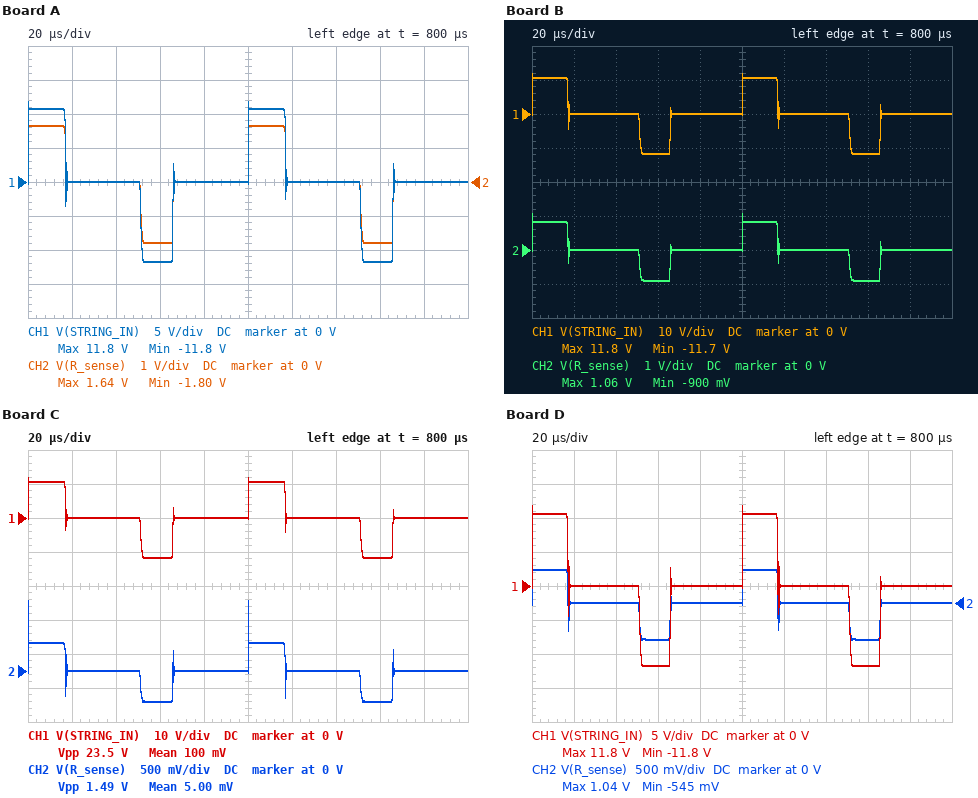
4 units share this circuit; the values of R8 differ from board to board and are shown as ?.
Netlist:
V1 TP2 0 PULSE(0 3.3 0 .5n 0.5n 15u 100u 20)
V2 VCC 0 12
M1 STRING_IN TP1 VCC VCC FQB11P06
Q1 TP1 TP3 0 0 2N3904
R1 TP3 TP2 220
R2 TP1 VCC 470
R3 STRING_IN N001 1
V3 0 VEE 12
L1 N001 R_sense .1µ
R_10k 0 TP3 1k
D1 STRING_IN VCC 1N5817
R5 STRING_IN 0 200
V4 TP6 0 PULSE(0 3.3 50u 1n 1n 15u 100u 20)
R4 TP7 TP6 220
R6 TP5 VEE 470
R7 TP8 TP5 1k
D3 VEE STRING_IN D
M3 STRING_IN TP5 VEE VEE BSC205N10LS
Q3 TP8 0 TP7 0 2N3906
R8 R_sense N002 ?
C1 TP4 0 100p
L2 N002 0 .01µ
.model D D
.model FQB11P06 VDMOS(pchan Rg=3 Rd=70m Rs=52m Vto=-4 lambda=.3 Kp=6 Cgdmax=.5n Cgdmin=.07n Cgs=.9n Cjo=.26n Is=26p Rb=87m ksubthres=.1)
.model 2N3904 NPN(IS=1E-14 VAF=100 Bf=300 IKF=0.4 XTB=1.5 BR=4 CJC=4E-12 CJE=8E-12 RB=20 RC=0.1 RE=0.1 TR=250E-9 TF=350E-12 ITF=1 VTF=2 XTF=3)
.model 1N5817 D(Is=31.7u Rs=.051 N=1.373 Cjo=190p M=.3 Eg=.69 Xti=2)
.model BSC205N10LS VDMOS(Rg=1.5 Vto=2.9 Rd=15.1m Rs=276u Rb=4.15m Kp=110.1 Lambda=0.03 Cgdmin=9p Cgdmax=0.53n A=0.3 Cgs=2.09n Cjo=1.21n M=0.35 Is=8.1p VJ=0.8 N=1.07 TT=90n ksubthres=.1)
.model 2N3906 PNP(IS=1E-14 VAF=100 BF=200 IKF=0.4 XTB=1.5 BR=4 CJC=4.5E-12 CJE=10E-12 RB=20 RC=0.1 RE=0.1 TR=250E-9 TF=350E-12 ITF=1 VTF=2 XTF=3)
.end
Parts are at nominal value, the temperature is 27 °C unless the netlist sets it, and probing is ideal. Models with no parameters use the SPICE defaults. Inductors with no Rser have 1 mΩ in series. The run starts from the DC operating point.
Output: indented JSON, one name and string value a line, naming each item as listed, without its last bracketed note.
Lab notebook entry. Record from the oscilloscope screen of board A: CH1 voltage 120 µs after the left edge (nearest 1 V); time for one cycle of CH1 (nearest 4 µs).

{
  "CH1 voltage 120 µs after the left edge": "0 V",
  "time for one cycle of CH1": "100 µs"
}
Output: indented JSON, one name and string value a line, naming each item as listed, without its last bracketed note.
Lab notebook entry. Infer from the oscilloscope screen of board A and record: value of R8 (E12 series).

{
  "value of R8": "0.18 Ω"
}
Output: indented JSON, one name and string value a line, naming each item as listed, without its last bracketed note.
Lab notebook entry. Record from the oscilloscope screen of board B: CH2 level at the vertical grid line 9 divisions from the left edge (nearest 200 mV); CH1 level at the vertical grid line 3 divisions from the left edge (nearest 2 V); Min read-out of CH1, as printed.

{
  "CH2 level at the vertical grid line 9 divisions from the left edge": "0 V",
  "CH1 level at the vertical grid line 3 divisions from the left edge": "-12 V",
  "Min read-out of CH1, as printed": "-11.7 V"
}
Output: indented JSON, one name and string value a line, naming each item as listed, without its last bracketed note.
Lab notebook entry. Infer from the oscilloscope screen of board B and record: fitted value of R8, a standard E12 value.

{
  "fitted value of R8, a standard E12 value": "0.082 Ω"
}
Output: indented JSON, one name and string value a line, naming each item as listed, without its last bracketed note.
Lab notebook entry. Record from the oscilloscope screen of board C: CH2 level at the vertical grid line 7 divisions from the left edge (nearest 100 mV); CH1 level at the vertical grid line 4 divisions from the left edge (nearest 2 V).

{
  "CH2 level at the vertical grid line 7 divisions from the left edge": "0 V",
  "CH1 level at the vertical grid line 4 divisions from the left edge": "0 V"
}
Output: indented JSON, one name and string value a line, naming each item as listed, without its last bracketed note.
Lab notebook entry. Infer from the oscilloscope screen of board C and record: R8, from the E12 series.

{
  "R8, from the E12 series": "0.039 Ω"
}
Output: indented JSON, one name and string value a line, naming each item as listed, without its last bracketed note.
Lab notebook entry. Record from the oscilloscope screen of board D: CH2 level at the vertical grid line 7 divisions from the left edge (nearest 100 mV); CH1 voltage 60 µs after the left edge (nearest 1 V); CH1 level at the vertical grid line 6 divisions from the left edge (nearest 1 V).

{
  "CH2 level at the vertical grid line 7 divisions from the left edge": "0 V",
  "CH1 voltage 60 µs after the left edge": "-12 V",
  "CH1 level at the vertical grid line 6 divisions from the left edge": "0 V"
}
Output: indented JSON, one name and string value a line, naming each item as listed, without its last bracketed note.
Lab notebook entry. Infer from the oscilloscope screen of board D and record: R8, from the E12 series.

{
  "R8, from the E12 series": "0.047 Ω"
}
